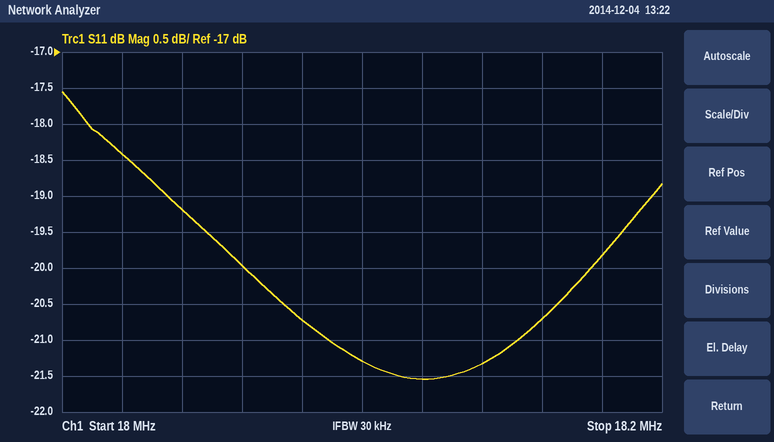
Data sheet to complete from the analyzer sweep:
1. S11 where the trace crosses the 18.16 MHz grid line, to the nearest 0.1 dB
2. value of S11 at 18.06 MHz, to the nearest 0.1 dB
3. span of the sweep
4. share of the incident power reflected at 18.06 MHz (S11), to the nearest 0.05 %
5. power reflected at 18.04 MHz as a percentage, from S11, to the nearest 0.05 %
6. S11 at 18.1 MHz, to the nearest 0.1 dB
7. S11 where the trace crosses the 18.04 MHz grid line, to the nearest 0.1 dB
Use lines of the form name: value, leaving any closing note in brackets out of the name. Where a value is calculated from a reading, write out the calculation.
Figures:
S11 where the trace crosses the 18.16 MHz grid line, to the nearest 0.1 dB: -20.7 dB
value of S11 at 18.06 MHz, to the nearest 0.1 dB: -20.0 dB
span of the sweep: 200 kHz
share of the incident power reflected at 18.06 MHz (S11), to the nearest 0.05 %: 10^(-20/10) ≈ 1.00 %
power reflected at 18.04 MHz as a percentage, from S11, to the nearest 0.05 %: 10^(-19.2/10) ≈ 1.20 %
S11 at 18.1 MHz, to the nearest 0.1 dB: -21.3 dB
S11 where the trace crosses the 18.04 MHz grid line, to the nearest 0.1 dB: -19.2 dB
